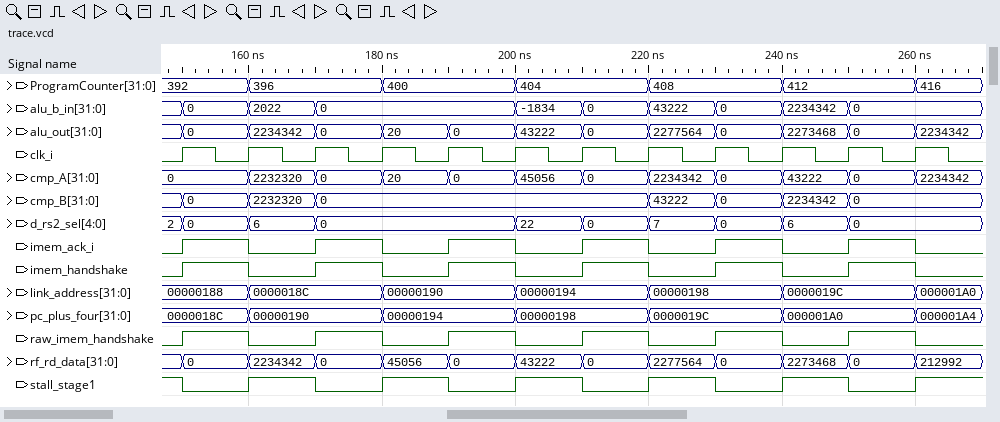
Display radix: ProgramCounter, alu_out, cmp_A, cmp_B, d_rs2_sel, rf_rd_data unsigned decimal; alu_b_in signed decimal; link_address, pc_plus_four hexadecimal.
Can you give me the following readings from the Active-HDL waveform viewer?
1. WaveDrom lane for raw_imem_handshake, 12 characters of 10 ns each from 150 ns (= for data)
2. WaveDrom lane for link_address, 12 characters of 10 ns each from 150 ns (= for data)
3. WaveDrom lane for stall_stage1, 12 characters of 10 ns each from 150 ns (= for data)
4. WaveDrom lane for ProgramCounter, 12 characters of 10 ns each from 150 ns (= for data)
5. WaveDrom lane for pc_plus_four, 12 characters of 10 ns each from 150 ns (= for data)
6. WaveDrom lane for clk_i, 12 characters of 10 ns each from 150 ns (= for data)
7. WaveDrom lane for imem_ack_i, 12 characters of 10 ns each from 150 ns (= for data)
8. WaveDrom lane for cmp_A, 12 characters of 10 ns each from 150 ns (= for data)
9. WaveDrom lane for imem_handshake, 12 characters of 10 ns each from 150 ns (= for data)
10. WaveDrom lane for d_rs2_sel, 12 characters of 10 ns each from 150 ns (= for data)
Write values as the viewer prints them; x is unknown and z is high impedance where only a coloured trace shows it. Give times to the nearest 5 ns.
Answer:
{name: 'raw_imem_handshake', wave: '101010101010'}
{name: 'link_address', wave: '==.=.=.=.=.=', data: '00000188 0000018C 00000190 00000194 00000198 0000019C 000001A0'}
{name: 'stall_stage1', wave: '010101010101'}
{name: 'ProgramCounter', wave: '==.=.=.=.=.=', data: '392 396 400 404 408 412 416'}
{name: 'pc_plus_four', wave: '==.=.=.=.=.=', data: '0000018C 00000190 00000194 00000198 0000019C 000001A0 000001A4'}
{name: 'clk_i', wave: 'p...........'}
{name: 'imem_ack_i', wave: '101010101010'}
{name: 'cmp_A', wave: '============', data: '0 2232320 0 20 0 45056 0 2234342 0 43222 0 2234342'}
{name: 'imem_handshake', wave: '101010101010'}
{name: 'd_rs2_sel', wave: '===..======.', data: '0 6 0 22 0 7 0 6 0'}
